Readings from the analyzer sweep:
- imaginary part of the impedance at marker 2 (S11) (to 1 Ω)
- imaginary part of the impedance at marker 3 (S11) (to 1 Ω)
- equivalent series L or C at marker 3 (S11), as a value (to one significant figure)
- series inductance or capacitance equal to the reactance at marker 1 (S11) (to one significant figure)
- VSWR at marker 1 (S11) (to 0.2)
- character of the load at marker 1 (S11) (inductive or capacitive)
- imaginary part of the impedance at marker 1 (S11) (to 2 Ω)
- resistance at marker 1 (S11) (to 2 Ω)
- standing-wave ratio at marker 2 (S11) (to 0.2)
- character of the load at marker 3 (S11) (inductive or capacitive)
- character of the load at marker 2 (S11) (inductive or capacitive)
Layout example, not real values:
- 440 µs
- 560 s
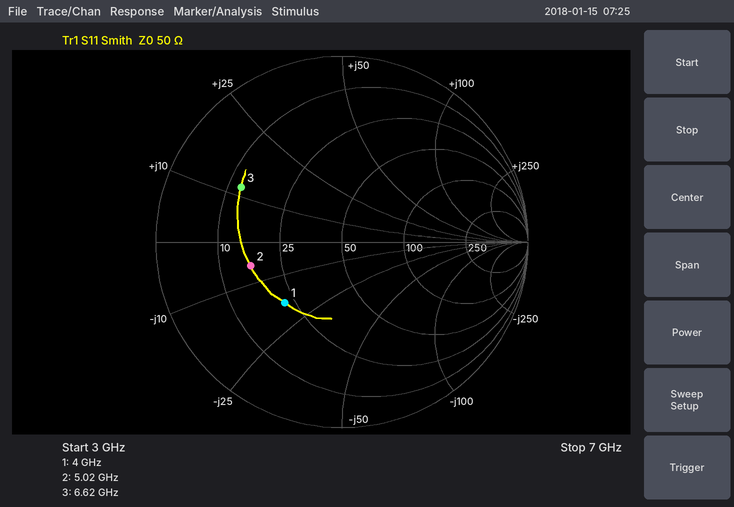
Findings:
- -6 Ω
- +12 Ω
- 300 pH
- 2 pF
- 2.6
- capacitive
- -18 Ω
- 22 Ω
- 3.0
- inductive
- capacitive
